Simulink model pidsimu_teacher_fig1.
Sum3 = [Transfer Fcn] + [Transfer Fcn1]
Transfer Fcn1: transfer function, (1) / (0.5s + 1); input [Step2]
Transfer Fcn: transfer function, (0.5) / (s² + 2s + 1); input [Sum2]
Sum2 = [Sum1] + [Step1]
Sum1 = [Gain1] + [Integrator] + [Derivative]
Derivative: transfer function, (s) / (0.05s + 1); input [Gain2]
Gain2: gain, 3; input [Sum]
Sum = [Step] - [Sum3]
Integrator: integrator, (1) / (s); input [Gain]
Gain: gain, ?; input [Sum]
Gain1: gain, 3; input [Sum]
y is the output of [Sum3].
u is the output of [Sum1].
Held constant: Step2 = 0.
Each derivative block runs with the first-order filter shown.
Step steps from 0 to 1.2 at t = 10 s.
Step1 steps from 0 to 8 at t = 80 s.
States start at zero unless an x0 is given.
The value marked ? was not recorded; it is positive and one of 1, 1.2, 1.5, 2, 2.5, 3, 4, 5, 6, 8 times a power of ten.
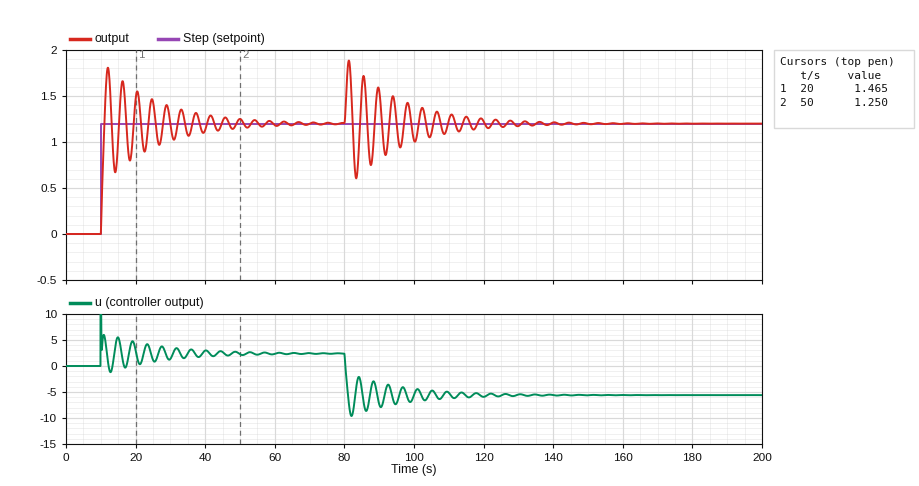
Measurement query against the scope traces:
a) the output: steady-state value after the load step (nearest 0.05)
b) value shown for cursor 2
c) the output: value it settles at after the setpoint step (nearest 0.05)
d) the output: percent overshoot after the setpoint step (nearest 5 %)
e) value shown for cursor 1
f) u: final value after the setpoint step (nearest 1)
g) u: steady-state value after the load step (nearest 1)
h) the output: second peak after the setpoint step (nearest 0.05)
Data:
1.20
1.250
1.20
50 %
1.465
2
-6
1.65
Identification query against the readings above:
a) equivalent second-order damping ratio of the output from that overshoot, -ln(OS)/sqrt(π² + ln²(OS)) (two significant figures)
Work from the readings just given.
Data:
0.22
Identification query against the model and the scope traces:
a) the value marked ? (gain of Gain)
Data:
15
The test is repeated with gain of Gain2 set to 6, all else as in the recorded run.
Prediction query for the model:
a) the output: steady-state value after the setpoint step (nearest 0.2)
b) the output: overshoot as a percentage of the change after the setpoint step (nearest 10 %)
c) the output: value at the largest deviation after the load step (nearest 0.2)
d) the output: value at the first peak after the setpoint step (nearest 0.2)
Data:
1.2
30 %
1.8
1.6
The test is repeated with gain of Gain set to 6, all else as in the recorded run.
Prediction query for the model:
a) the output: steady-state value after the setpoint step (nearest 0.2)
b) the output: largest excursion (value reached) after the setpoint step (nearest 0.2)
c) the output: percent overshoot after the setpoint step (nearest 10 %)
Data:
1.2
1.4
20 %
